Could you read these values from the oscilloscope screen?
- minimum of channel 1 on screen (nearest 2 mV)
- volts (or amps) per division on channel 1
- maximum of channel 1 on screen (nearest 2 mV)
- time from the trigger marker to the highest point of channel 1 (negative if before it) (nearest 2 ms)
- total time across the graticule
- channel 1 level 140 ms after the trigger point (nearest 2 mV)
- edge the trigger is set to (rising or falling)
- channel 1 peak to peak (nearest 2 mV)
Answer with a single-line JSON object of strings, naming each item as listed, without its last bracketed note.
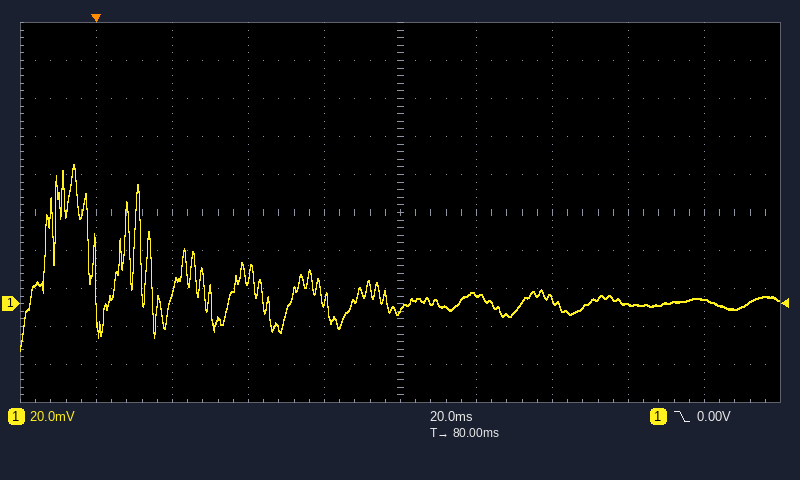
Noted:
{"minimum of channel 1 on screen": "-24 mV", "volts (or amps) per division on channel 1": "20 mV", "maximum of channel 1 on screen": "74 mV", "time from the trigger marker to the highest point of channel 1 (negative if before it)": "-6 ms", "total time across the graticule": "200 ms", "channel 1 level 140 ms after the trigger point": "0 mV", "edge the trigger is set to": "falling", "channel 1 peak to peak": "98 mV"}
